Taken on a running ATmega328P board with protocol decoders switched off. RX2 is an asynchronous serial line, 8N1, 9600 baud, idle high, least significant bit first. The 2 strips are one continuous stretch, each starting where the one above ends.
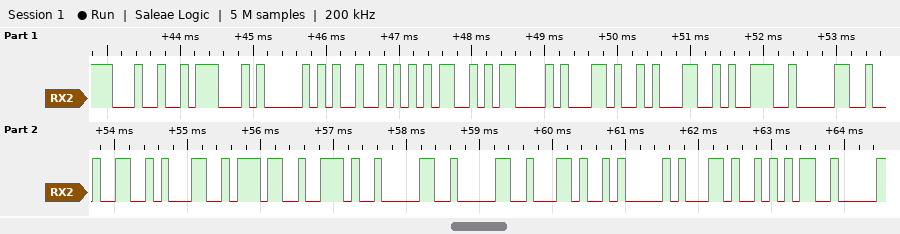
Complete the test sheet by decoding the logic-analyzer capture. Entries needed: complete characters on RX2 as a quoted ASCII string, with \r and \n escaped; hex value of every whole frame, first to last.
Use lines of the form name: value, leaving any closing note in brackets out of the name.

complete characters on RX2 as a quoted ASCII string, with \r and \n escaped: "$GPRMC,190217.00,A,5"
hex value of every whole frame, first to last: 24 47 50 52 4D 43 2C 31 39 30 32 31 37 2E 30 30 2C 41 2C 35
